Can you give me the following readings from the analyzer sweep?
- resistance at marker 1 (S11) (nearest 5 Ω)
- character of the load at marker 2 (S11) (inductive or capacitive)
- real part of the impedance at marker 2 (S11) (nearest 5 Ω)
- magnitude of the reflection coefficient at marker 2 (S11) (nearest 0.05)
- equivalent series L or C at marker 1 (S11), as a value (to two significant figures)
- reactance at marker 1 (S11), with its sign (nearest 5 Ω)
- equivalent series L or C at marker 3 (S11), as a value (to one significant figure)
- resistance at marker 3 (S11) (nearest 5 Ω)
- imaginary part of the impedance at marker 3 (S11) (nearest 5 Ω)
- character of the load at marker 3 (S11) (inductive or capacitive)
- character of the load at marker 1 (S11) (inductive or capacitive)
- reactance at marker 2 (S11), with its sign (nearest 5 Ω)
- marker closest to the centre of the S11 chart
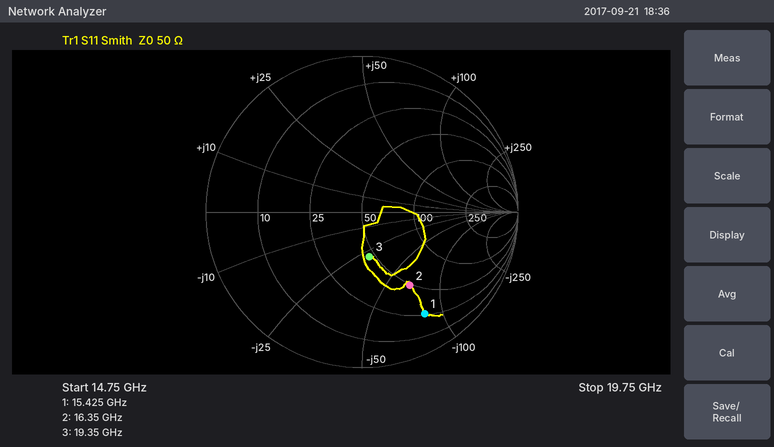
25 Ω
capacitive
50 Ω
0.55
120 fF
-85 Ω
300 fF
45 Ω
-30 Ω
capacitive
capacitive
-65 Ω
marker 3
